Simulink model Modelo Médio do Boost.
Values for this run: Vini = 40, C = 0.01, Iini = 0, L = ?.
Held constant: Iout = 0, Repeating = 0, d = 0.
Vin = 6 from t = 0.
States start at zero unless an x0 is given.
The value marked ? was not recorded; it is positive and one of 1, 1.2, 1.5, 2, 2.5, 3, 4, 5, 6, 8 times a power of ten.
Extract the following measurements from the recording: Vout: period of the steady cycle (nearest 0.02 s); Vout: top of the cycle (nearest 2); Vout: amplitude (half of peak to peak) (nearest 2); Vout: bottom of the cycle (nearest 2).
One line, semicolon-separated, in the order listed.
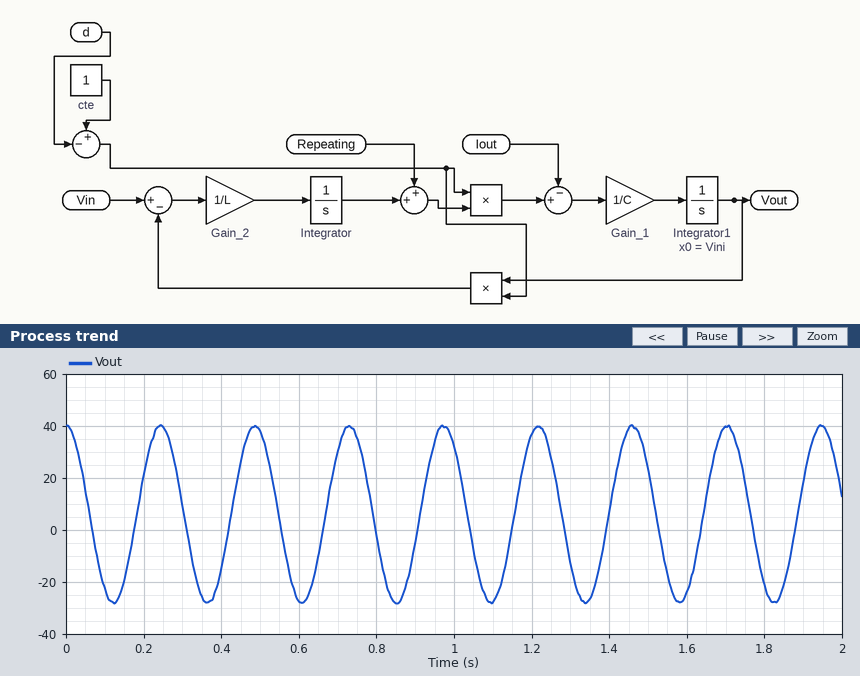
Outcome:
0.24 s; 40; 34; -28
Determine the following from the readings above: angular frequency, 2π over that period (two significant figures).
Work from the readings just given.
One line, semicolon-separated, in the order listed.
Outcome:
26 rad/s
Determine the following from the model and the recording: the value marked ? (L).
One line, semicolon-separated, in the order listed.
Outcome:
0.15
